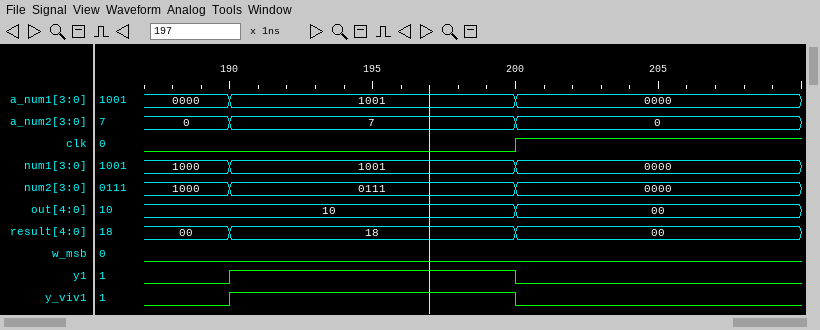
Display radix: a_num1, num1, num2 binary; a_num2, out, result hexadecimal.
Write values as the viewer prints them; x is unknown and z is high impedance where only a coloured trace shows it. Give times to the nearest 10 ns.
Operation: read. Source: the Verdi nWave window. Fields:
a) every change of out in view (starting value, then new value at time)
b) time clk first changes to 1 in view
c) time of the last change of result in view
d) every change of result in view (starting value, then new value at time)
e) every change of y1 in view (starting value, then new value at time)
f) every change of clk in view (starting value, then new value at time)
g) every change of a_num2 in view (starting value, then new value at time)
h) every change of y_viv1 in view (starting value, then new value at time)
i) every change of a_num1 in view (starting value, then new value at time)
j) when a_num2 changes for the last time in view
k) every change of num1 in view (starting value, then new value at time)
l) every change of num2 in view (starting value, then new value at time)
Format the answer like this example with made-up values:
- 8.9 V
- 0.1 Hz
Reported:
- 10, 00 at 200 ns
- 200 ns
- 200 ns
- 00, 18 at 190 ns, 00 at 200 ns
- 0, 1 at 190 ns, 0 at 200 ns
- 0, 1 at 200 ns
- 0, 7 at 190 ns, 0 at 200 ns
- 0, 1 at 190 ns, 0 at 200 ns
- 0000, 1001 at 190 ns, 0000 at 200 ns
- 200 ns
- 1000, 1001 at 190 ns, 0000 at 200 ns
- 1000, 0111 at 190 ns, 0000 at 200 ns
